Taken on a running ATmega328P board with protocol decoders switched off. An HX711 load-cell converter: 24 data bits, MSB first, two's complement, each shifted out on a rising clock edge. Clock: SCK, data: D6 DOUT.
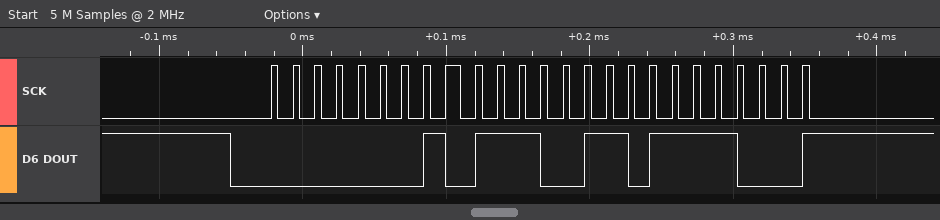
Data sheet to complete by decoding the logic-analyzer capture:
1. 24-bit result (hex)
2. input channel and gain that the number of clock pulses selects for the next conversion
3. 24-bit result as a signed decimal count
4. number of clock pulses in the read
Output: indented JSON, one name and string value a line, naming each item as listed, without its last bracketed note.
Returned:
{
  "24-bit result": "0x017378",
  "input channel and gain that the number of clock pulses selects for the next conversion": "channel A, gain 128",
  "24-bit result as a signed decimal count": "95096",
  "number of clock pulses in the read": "25"
}
